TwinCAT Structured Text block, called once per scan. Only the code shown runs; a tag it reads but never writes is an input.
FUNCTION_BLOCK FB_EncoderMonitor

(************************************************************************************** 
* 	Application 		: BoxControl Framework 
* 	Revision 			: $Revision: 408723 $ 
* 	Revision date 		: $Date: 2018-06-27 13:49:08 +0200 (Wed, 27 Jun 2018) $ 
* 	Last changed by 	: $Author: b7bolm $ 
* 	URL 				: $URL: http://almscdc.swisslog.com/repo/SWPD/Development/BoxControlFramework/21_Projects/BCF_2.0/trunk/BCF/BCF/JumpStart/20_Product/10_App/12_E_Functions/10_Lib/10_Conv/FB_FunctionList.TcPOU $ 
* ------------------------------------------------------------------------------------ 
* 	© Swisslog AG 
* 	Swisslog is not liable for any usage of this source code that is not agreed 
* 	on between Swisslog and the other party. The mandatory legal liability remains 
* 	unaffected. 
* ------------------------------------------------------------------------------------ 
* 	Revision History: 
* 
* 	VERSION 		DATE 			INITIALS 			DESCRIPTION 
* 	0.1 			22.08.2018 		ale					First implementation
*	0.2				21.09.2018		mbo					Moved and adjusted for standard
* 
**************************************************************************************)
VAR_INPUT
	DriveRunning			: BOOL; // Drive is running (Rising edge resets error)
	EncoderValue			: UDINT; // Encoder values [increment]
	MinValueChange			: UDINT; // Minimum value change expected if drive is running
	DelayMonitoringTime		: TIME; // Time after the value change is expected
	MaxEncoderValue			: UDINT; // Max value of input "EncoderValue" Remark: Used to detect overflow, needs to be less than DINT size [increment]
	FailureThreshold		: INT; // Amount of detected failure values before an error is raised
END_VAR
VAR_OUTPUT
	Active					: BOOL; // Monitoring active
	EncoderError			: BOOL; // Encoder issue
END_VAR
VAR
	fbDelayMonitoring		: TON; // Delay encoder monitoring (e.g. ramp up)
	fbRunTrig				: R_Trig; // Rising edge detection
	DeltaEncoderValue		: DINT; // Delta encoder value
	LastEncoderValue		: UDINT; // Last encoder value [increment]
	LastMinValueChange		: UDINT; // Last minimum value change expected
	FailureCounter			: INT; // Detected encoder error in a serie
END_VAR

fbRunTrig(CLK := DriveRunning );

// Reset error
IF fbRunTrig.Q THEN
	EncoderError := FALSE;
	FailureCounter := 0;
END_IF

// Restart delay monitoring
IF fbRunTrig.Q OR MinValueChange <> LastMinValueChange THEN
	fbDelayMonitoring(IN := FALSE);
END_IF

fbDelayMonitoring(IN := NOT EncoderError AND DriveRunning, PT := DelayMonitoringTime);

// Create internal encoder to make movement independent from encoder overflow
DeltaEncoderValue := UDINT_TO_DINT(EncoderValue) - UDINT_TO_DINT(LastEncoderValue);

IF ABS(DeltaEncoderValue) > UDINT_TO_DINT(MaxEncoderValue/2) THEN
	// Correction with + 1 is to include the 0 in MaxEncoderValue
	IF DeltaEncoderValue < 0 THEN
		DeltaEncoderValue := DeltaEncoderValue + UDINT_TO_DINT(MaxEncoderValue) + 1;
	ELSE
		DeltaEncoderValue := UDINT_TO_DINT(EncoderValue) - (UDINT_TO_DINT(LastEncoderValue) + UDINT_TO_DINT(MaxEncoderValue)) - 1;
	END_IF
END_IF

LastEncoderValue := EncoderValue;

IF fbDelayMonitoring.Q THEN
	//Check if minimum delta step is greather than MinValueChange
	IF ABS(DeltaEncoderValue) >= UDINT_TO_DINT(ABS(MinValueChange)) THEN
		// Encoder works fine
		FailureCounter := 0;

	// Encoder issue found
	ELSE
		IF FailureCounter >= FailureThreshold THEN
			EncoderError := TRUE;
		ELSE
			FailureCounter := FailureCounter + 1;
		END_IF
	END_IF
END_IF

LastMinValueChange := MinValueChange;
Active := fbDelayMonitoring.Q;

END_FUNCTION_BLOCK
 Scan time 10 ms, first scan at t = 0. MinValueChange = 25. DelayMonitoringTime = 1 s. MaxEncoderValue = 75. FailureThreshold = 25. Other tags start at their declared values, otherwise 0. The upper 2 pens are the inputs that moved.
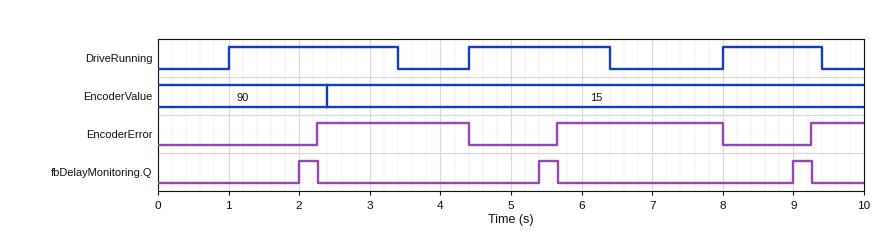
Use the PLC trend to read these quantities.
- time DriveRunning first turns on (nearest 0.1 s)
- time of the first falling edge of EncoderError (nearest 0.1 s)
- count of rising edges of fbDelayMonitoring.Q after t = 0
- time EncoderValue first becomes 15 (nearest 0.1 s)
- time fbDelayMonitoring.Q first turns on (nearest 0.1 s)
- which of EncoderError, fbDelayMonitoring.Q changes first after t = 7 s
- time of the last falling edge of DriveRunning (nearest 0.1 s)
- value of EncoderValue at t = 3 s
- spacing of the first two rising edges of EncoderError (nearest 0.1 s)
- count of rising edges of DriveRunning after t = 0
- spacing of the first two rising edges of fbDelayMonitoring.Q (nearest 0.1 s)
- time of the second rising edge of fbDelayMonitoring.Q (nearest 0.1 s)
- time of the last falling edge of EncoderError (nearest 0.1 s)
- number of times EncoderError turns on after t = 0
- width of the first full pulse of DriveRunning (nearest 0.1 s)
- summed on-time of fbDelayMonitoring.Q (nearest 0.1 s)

1.0 s
4.4 s
3
2.4 s
2.0 s
EncoderError
9.4 s
15
3.4 s
3
3.4 s
5.4 s
8.0 s
3
2.4 s
0.8 s
